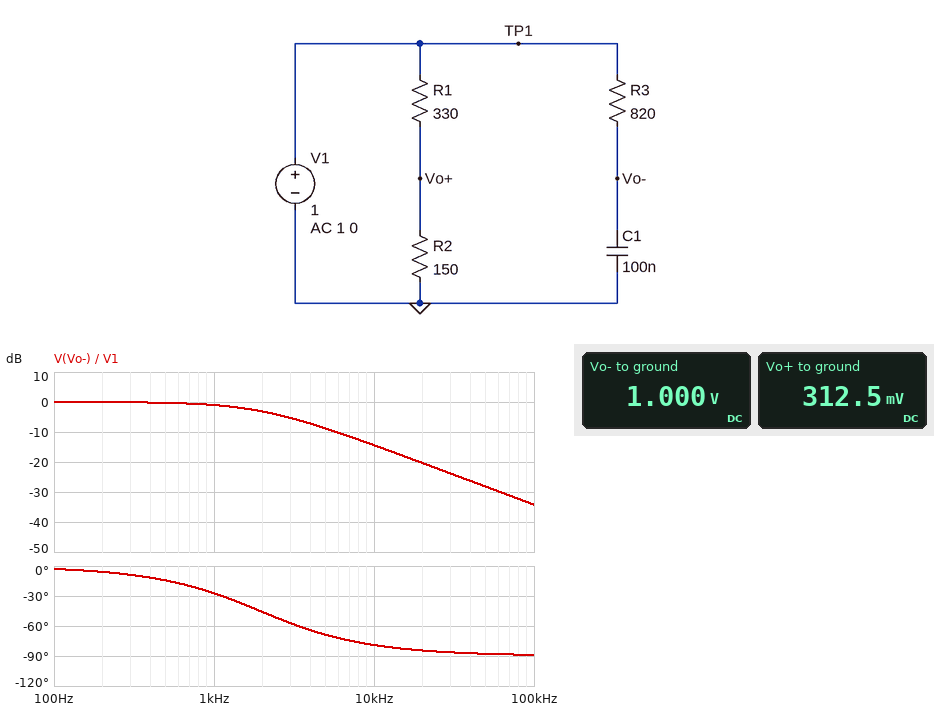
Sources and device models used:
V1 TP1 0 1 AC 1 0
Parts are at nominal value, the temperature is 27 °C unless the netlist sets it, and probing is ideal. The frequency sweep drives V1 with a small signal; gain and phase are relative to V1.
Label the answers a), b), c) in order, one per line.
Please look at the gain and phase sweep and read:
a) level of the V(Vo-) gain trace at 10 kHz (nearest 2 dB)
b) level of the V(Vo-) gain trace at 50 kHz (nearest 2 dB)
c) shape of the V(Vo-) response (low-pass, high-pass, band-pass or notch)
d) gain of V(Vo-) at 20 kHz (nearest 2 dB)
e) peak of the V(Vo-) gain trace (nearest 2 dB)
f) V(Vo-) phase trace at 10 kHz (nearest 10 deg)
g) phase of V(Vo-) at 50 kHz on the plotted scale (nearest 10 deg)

a) -14 dB
b) -28 dB
c) low-pass
d) -20 dB
e) 0 dB
f) -80 deg
g) -90 deg
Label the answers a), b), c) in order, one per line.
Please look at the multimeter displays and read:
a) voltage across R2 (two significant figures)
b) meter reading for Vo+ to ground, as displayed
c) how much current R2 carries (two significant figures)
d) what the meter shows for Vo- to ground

a) 310 mV
b) 312.5 mV
c) 2.1 mA
d) 1.000 V
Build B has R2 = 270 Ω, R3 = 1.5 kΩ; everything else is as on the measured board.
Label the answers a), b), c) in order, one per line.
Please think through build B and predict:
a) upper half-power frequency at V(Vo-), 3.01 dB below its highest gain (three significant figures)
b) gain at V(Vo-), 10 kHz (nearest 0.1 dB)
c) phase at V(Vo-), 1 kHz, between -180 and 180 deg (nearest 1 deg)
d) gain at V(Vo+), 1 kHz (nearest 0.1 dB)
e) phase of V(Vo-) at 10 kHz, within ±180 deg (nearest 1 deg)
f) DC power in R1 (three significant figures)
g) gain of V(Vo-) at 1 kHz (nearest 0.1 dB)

a) 1.06 kHz
b) -19.5 dB
c) -43 deg
d) -6.9 dB
e) -84 deg
f) 917 µW
g) -2.8 dB
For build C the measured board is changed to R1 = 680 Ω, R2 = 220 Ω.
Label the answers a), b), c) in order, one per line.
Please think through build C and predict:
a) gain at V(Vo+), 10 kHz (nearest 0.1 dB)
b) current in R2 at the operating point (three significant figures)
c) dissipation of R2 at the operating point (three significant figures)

a) -12.2 dB
b) 1.11 mA
c) 272 µW
